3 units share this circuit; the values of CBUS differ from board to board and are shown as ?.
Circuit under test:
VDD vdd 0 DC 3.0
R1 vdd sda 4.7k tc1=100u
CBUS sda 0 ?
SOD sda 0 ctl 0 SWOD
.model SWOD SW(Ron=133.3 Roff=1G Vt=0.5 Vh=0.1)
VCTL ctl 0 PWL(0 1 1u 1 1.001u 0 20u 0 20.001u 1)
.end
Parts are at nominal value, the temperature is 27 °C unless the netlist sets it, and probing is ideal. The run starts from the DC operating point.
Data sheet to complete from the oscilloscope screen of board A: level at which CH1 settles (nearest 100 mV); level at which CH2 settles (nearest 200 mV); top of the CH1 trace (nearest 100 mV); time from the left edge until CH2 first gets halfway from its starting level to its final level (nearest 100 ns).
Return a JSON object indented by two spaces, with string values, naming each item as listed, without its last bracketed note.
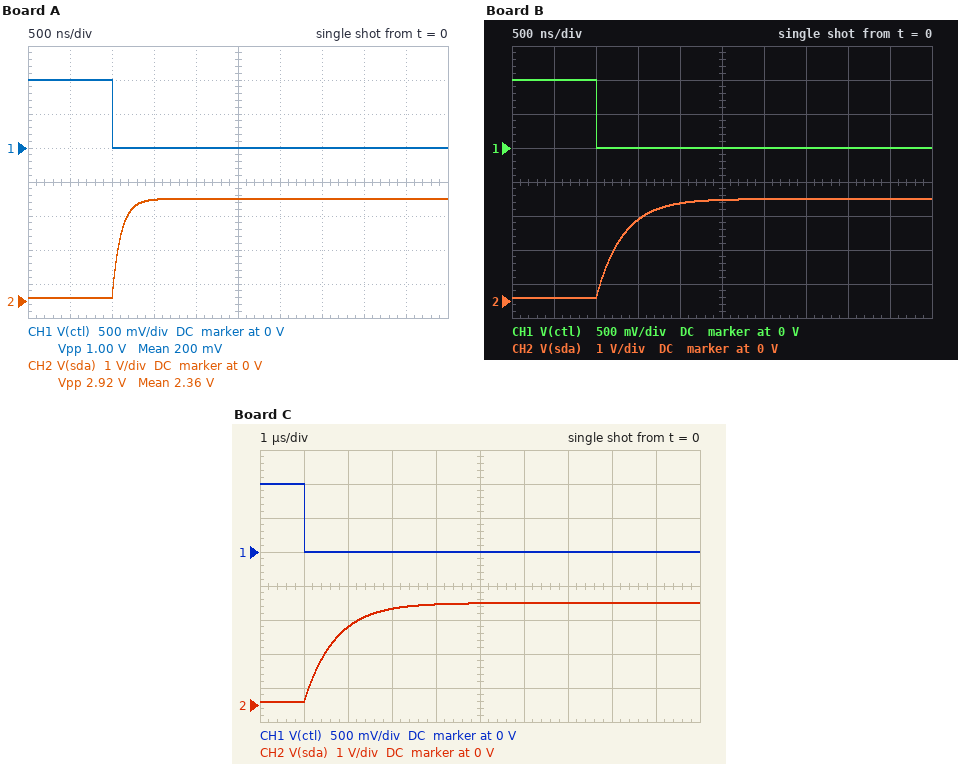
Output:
{
  "level at which CH1 settles": "0 V",
  "level at which CH2 settles": "3.0 V",
  "top of the CH1 trace": "1.0 V",
  "time from the left edge until CH2 first gets halfway from its starting level to its final level": "1.1 µs"
}
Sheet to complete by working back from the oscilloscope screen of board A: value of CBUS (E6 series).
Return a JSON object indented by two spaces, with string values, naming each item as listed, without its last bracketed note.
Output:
{
  "value of CBUS": "22 pF"
}
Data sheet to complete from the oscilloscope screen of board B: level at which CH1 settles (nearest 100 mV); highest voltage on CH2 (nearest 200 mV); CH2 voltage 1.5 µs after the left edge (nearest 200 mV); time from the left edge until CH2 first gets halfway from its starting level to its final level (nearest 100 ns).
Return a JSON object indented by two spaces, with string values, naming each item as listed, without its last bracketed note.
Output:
{
  "level at which CH1 settles": "0 V",
  "highest voltage on CH2": "3.0 V",
  "CH2 voltage 1.5 µs after the left edge": "2.4 V",
  "time from the left edge until CH2 first gets halfway from its starting level to its final level": "1.2 µs"
}
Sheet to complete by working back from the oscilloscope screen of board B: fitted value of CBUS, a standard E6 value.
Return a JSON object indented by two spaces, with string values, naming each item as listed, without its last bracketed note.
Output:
{
  "fitted value of CBUS, a standard E6 value": "68 pF"
}
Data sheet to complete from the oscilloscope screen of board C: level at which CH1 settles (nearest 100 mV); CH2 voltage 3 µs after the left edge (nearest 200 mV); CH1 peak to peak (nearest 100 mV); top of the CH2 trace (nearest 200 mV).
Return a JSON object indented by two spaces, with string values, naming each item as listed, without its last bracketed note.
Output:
{
  "level at which CH1 settles": "0 V",
  "CH2 voltage 3 µs after the left edge": "2.8 V",
  "CH1 peak to peak": "1.0 V",
  "top of the CH2 trace": "3.0 V"
}
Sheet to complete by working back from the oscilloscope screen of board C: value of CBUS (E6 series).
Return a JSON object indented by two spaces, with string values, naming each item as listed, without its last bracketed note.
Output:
{
  "value of CBUS": "150 pF"
}
